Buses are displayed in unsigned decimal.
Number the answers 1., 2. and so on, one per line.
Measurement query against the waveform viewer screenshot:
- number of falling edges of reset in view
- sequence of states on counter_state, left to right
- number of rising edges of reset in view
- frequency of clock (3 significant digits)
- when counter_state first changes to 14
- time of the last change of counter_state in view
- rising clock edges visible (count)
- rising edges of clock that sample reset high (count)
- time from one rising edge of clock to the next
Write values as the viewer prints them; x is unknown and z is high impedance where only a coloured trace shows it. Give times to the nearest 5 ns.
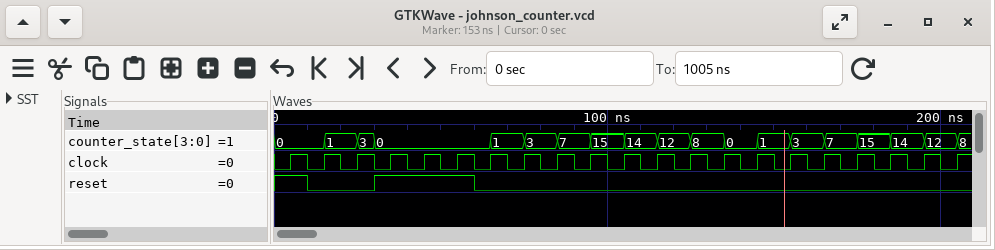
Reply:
1. 2
2. 0, 1, 3, 0, 1, 3, 7, 15, 14, 12, 8, 0, 1, 3, 7, 15, 14, 12, 8
3. 1
4. 100 MHz
5. 105 ns
6. 205 ns
7. 21
8. 4
9. 10 ns
